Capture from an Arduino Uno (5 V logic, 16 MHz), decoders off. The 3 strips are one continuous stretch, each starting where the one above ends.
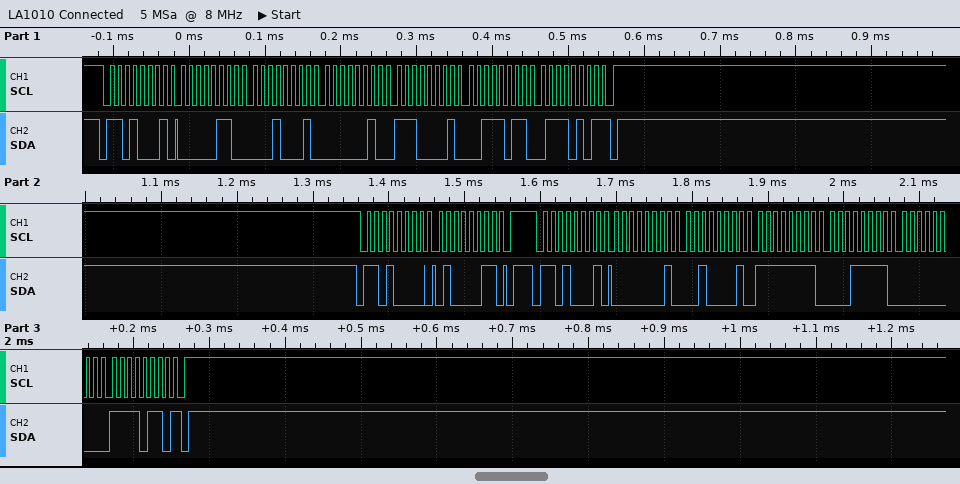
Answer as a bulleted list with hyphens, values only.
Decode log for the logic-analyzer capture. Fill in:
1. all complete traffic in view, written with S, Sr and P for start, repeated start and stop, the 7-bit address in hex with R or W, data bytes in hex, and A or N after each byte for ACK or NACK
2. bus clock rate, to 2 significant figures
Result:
- S 68R A 06 A 11 A 02 A E1 A 3B A 75 N P S 68W A 43 A P S 68R A 01 A 21 A FF A 1F A 00 A F6 N P
- 100 kHz
